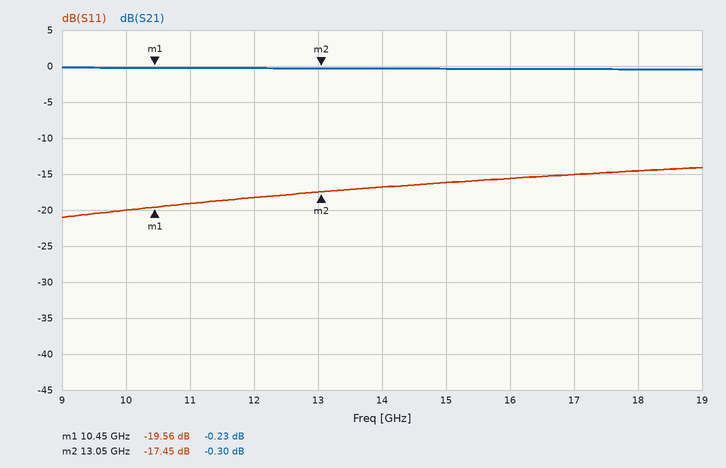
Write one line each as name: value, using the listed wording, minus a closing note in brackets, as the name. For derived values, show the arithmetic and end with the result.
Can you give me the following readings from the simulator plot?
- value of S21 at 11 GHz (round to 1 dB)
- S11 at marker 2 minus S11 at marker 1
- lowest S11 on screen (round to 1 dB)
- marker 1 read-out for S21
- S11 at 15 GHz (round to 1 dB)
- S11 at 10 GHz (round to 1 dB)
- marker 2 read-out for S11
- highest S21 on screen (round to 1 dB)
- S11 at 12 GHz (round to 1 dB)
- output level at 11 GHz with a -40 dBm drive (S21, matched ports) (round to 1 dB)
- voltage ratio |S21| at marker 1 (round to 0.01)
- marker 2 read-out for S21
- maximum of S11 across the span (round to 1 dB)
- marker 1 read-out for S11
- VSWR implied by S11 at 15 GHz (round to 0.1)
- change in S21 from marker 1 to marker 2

value of S21 at 11 GHz: 0 dB
S11 at marker 2 minus S11 at marker 1: -17.45 − (-19.56) = 2.11 dB
lowest S11 on screen: -21 dB
marker 1 read-out for S21: -0.23 dB
S11 at 15 GHz: -16 dB
S11 at 10 GHz: -20 dB
marker 2 read-out for S11: -17.45 dB
highest S21 on screen: 0 dB
S11 at 12 GHz: -18 dB
output level at 11 GHz with a -40 dBm drive (S21, matched ports): -40 dBm + (0 dB) = -40 dBm
voltage ratio |S21| at marker 1: 10^(-0.23/20) ≈ 0.97
marker 2 read-out for S21: -0.30 dB
maximum of S11 across the span: -14 dB
marker 1 read-out for S11: -19.56 dB
VSWR implied by S11 at 15 GHz: |Γ| = 10^(-16/20) = 0.1585; VSWR = (1 + 0.1585)/(1 − 0.1585) ≈ 1.4
change in S21 from marker 1 to marker 2: -0.3 − (-0.23) = -0.07 dB
